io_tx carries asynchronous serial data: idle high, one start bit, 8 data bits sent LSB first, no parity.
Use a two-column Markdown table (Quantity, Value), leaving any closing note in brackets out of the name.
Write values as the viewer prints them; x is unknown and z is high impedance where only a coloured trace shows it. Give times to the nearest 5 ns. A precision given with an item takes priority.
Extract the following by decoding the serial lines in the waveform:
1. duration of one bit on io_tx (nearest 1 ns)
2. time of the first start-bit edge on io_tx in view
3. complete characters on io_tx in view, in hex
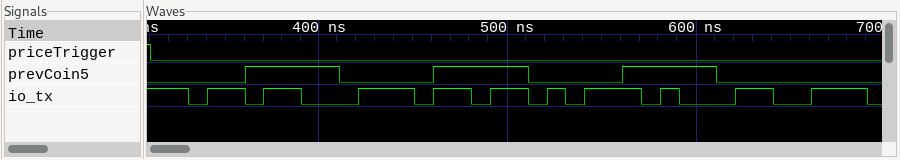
| Quantity | Value |
|---|---|
| duration of one bit on io_tx | 10 ns |
| time of the first start-bit edge on io_tx in view | 330 ns |
| complete characters on io_tx in view, in hex | 1B, 5B, 31 |
